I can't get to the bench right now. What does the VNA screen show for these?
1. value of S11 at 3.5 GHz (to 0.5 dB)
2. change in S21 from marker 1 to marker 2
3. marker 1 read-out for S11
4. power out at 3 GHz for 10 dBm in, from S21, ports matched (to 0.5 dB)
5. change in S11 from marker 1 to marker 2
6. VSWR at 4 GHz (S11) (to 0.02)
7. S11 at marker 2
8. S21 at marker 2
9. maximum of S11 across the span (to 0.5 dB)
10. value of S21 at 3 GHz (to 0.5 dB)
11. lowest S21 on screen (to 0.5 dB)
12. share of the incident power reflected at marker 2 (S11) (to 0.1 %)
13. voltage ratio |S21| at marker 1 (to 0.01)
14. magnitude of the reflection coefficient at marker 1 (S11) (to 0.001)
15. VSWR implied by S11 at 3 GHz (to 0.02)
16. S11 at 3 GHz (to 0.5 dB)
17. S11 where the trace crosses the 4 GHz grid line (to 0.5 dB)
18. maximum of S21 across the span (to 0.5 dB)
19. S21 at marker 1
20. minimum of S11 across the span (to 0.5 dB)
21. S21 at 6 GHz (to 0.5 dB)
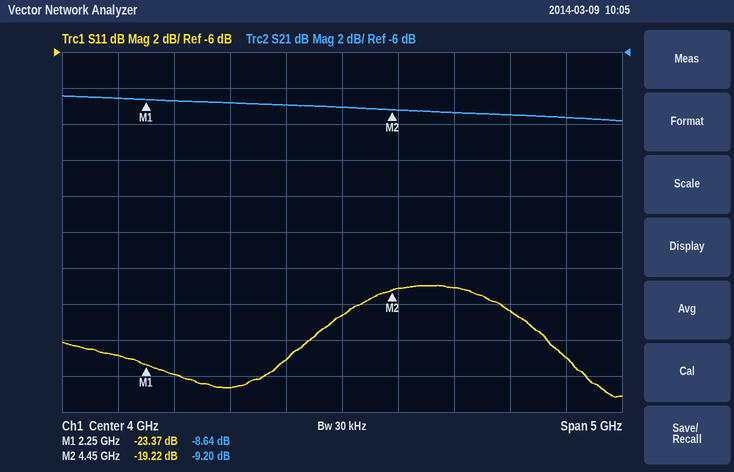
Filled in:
-23.0 dB
-0.56 dB
-23.37 dB
1.0 dBm
4.15 dB
1.20
-19.22 dB
-9.20 dB
-19.0 dB
-9.0 dB
-10.0 dB
1.2 %
0.37
0.068
1.12
-24.5 dB
-20.5 dB
-8.5 dB
-8.64 dB
-25.0 dB
-9.5 dB
